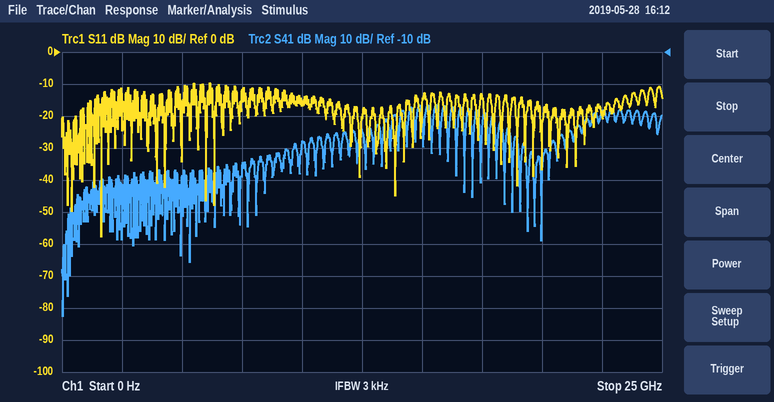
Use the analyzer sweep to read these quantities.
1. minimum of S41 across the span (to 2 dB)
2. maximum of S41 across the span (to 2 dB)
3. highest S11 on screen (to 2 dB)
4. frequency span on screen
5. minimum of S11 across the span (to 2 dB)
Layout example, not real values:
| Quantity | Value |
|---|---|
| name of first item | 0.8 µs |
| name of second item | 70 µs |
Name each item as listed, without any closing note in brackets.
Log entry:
| Quantity | Value |
|---|---|
| minimum of S41 across the span | -92 dB |
| maximum of S41 across the span | -26 dB |
| highest S11 on screen | -10 dB |
| frequency span on screen | 25 GHz |
| minimum of S11 across the span | -58 dB |
